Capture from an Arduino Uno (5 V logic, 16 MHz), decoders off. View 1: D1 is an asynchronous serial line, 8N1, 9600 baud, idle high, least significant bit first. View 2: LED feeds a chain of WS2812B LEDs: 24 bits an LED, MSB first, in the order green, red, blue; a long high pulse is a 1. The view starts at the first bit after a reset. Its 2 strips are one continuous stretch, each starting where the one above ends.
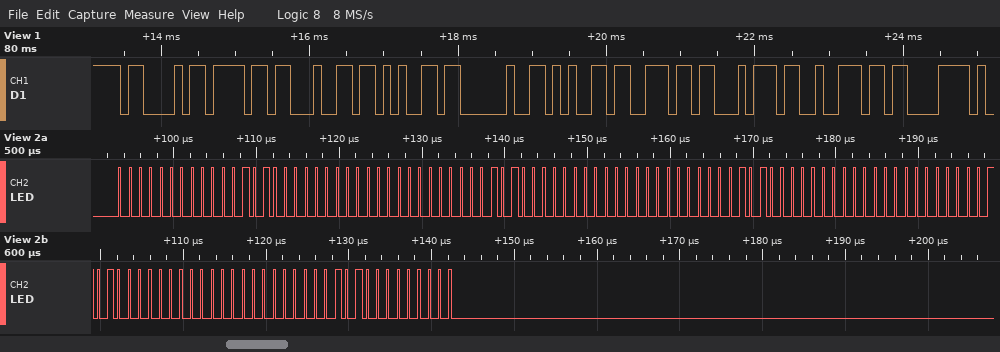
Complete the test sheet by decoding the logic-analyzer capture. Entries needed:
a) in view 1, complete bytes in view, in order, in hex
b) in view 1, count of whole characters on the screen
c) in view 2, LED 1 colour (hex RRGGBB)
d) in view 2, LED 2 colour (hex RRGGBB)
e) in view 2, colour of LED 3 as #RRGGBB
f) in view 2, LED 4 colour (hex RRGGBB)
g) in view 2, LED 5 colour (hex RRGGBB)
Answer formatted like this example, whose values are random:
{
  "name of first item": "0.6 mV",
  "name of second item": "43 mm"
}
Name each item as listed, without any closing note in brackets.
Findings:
{
  "in view 1, complete bytes in view, in order, in hex": "43 6F 64 65 20 65 6E 74 72 C3",
  "in view 1, count of whole characters on the screen": "10",
  "in view 2, LED 1 colour": "#0A0000",
  "in view 2, LED 2 colour": "#0A0000",
  "in view 2, colour of LED 3 as #RRGGBB": "#0A0000",
  "in view 2, LED 4 colour": "#0A0000",
  "in view 2, LED 5 colour": "#0A0000"
}
